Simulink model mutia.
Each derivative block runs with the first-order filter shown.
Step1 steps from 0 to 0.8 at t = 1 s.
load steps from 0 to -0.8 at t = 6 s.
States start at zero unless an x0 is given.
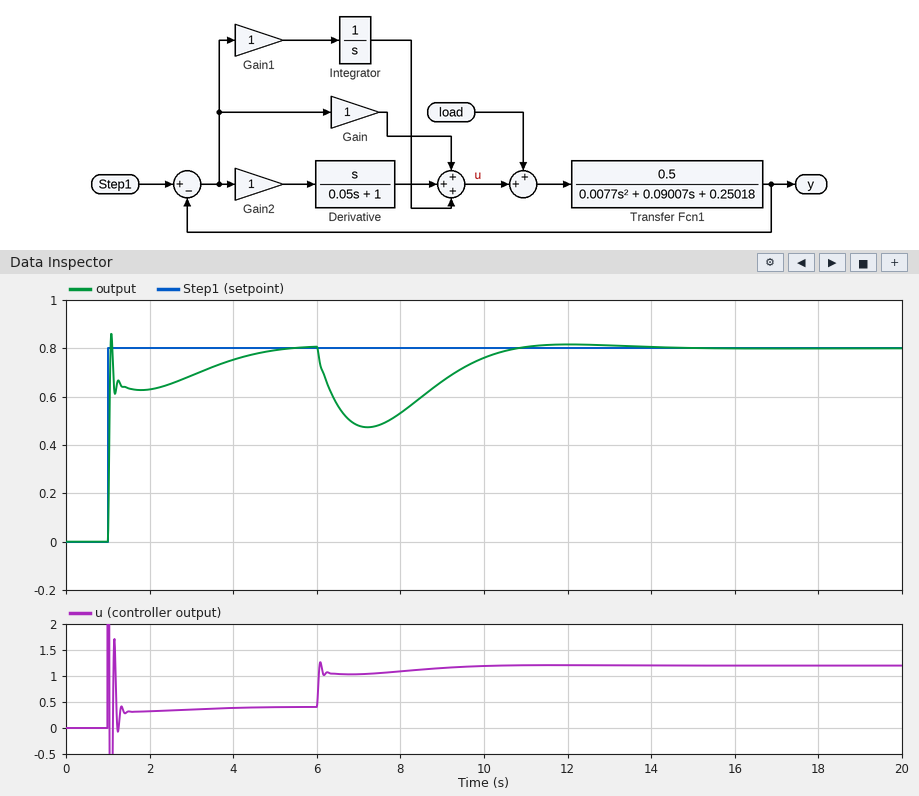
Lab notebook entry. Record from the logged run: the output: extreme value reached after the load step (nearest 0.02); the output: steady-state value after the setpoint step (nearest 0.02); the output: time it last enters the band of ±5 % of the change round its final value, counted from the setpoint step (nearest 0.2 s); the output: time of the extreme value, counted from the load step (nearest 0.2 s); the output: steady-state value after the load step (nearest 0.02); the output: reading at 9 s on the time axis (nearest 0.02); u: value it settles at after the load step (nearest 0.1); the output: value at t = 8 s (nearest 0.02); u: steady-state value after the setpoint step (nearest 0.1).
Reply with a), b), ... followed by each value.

a) 0.48
b) 0.80
c) 3.2 s
d) 1.2 s
e) 0.80
f) 0.66
g) 1.2
h) 0.54
i) 0.4
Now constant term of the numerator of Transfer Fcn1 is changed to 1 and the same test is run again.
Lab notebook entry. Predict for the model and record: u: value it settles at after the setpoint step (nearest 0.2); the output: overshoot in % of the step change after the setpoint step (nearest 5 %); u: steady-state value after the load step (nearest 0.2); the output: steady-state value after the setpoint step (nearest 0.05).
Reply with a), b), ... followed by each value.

a) 0.2
b) 30 %
c) 1.0
d) 0.80
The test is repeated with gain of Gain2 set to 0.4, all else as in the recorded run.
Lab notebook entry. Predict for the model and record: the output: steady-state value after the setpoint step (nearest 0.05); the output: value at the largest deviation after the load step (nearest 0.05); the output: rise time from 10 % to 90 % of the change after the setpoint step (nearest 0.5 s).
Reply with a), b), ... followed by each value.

a) 0.80
b) 0.40
c) 2.0 s
